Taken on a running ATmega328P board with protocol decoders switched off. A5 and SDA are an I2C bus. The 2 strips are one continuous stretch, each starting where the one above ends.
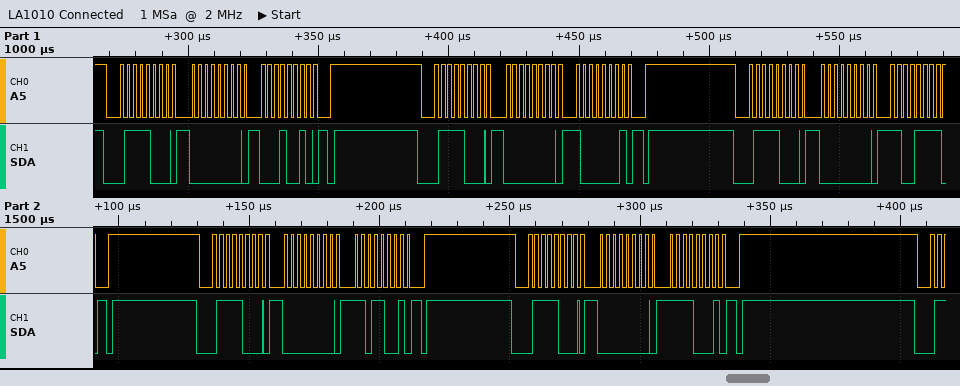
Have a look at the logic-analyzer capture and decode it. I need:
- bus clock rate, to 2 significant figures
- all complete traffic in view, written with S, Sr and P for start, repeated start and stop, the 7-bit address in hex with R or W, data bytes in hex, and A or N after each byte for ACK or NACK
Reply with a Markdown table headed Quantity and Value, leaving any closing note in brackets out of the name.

| Quantity | Value |
|---|---|
| bus clock rate, to 2 significant figures | 400 kHz |
| all complete traffic in view, written with S, Sr and P for start, repeated start and stop, the 7-bit address in hex with R or W, data bytes in hex, and A or N after each byte for ACK or NACK | S 3CW A 00 A 12 A P S 3CW A 00 A 81 A P S 3CW A 00 A CF A P S 3CW A 00 A D9 A P S 3CW A 00 A F1 A P |
